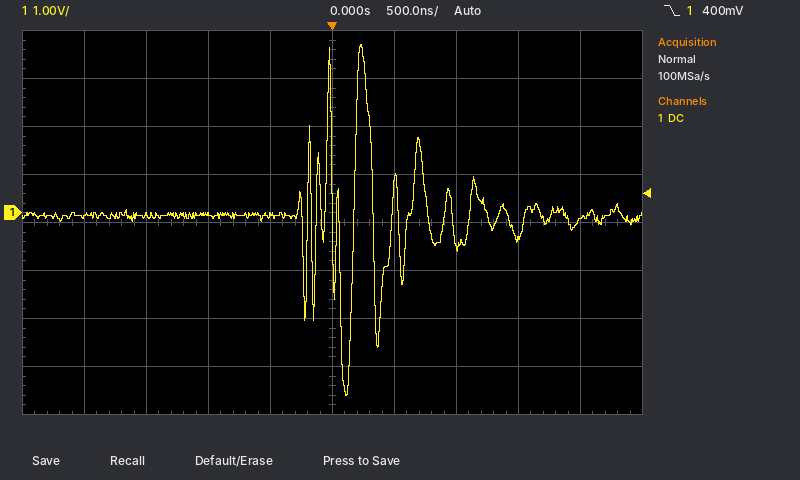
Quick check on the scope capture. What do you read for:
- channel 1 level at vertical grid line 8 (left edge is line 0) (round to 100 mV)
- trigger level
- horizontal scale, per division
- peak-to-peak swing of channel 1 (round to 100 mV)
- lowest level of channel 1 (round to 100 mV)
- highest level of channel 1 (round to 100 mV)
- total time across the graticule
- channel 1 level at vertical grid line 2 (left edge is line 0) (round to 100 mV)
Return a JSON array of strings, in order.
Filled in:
["-500 mV", "400 mV", "500 ns", "7.3 V", "-3.8 V", "3.5 V", "5 µs", "-100 mV"]
